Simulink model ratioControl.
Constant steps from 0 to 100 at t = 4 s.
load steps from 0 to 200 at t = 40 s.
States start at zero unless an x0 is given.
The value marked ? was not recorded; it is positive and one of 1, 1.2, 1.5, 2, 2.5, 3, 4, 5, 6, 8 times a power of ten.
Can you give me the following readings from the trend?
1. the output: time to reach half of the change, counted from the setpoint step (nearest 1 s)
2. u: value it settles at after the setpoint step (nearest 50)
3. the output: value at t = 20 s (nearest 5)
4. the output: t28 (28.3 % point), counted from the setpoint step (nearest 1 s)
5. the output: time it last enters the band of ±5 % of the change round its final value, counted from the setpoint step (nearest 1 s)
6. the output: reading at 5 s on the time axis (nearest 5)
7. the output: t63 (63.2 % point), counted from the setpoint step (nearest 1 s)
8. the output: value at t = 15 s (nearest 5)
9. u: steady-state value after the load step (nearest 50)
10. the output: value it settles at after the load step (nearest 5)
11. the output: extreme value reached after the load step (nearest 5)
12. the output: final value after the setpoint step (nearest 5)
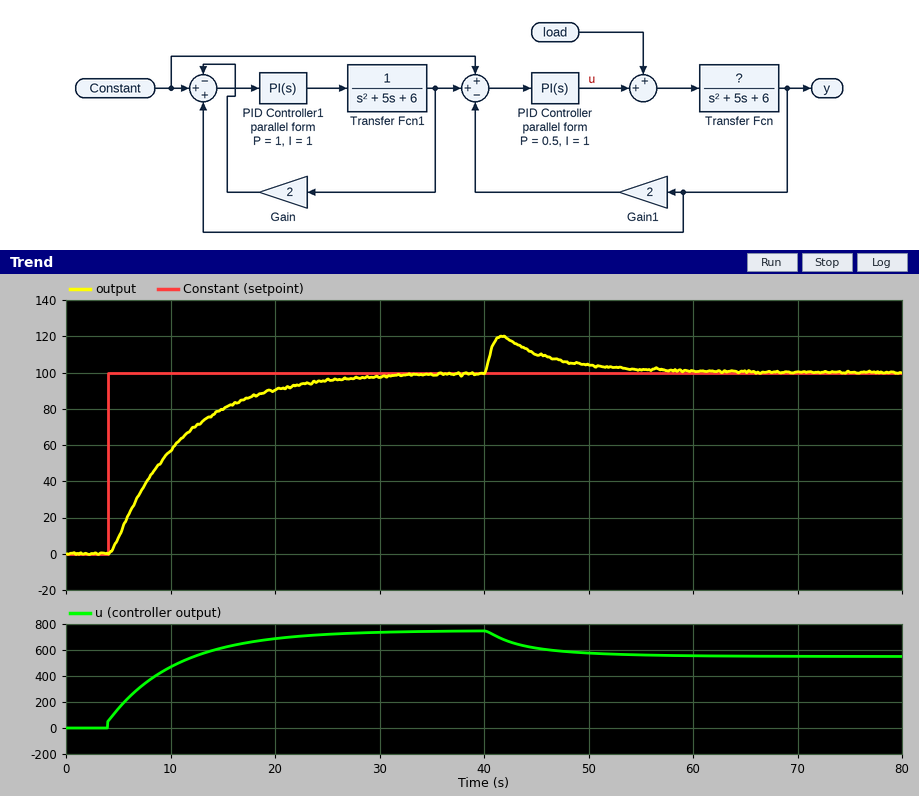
5 s
750
90
3 s
20 s
10
7 s
80
550
100
120
100
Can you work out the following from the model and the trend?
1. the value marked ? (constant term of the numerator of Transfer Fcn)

0.8
